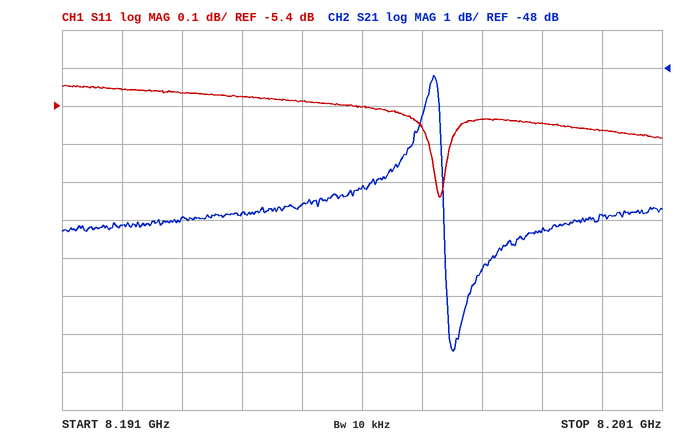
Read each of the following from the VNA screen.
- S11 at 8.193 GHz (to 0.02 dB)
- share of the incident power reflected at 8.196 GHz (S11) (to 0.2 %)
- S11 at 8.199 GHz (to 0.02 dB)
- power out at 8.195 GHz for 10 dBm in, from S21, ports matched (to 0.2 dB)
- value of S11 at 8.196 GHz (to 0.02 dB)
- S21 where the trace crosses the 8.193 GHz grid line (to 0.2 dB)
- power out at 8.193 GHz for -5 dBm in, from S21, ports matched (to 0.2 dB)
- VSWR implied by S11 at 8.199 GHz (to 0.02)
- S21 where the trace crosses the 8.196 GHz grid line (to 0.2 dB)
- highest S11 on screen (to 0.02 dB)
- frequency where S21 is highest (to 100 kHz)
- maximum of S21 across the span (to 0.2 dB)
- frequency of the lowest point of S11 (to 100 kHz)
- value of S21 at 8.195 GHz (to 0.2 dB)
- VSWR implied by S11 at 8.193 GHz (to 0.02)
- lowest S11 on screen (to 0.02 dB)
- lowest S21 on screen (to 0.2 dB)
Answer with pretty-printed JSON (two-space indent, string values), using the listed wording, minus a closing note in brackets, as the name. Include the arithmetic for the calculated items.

{
  "S11 at 8.193 GHz": "-5.36 dB",
  "share of the incident power reflected at 8.196 GHz (S11)": "10^(-5.4/10) ≈ 28.8 %",
  "S11 at 8.199 GHz": "-5.44 dB",
  "power out at 8.195 GHz for 10 dBm in, from S21, ports matched": "10 dBm + (-51.6 dB) = -41.6 dBm",
  "value of S11 at 8.196 GHz": "-5.40 dB",
  "S21 where the trace crosses the 8.193 GHz grid line": "-52.0 dB",
  "power out at 8.193 GHz for -5 dBm in, from S21, ports matched": "-5 dBm + (-52.0 dB) = -57.0 dBm",
  "VSWR implied by S11 at 8.199 GHz": "|Γ| = 10^(-5.44/20) = 0.5346; VSWR = (1 + 0.5346)/(1 − 0.5346) ≈ 3.30",
  "S21 where the trace crosses the 8.196 GHz grid line": "-51.2 dB",
  "highest S11 on screen": "-5.34 dB",
  "frequency where S21 is highest": "8.1972 GHz",
  "maximum of S21 across the span": "-48.2 dB",
  "frequency of the lowest point of S11": "8.1973 GHz",
  "value of S21 at 8.195 GHz": "-51.6 dB",
  "VSWR implied by S11 at 8.193 GHz": "|Γ| = 10^(-5.36/20) = 0.5395; VSWR = (1 + 0.5395)/(1 − 0.5395) ≈ 3.34",
  "lowest S11 on screen": "-5.64 dB",
  "lowest S21 on screen": "-55.4 dB"
}
